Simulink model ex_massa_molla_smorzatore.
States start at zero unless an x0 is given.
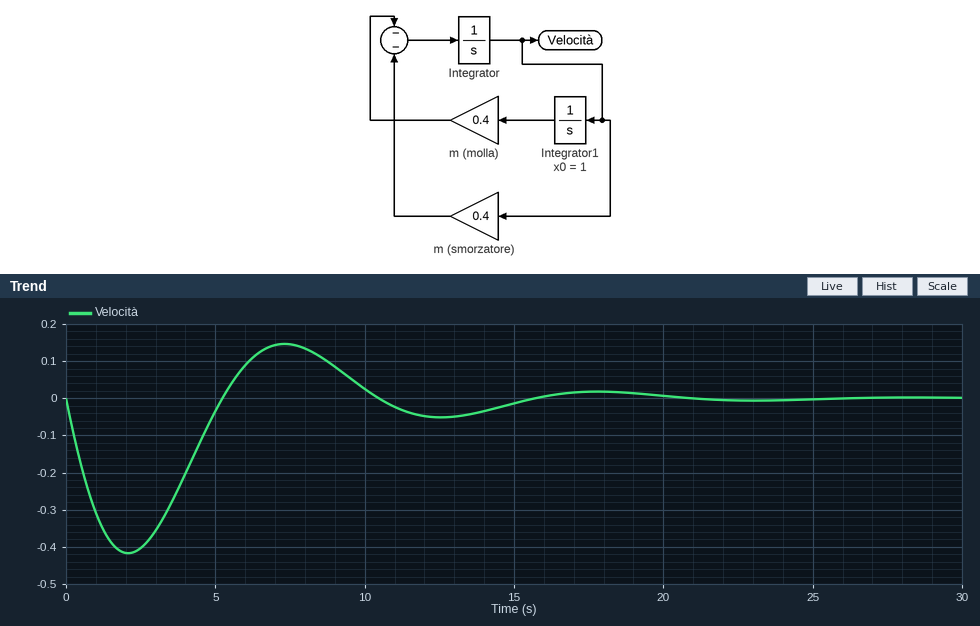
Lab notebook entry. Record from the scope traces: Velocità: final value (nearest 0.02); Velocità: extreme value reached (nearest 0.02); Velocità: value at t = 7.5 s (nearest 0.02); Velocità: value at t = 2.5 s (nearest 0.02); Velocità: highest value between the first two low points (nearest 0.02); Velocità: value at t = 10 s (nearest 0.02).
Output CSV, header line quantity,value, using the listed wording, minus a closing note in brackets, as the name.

quantity,value
Velocità: final value,0.00
Velocità: extreme value reached,-0.42
Velocità: value at t = 7.5 s,0.14
Velocità: value at t = 2.5 s,-0.40
Velocità: highest value between the first two low points,0.14
Velocità: value at t = 10 s,0.02
